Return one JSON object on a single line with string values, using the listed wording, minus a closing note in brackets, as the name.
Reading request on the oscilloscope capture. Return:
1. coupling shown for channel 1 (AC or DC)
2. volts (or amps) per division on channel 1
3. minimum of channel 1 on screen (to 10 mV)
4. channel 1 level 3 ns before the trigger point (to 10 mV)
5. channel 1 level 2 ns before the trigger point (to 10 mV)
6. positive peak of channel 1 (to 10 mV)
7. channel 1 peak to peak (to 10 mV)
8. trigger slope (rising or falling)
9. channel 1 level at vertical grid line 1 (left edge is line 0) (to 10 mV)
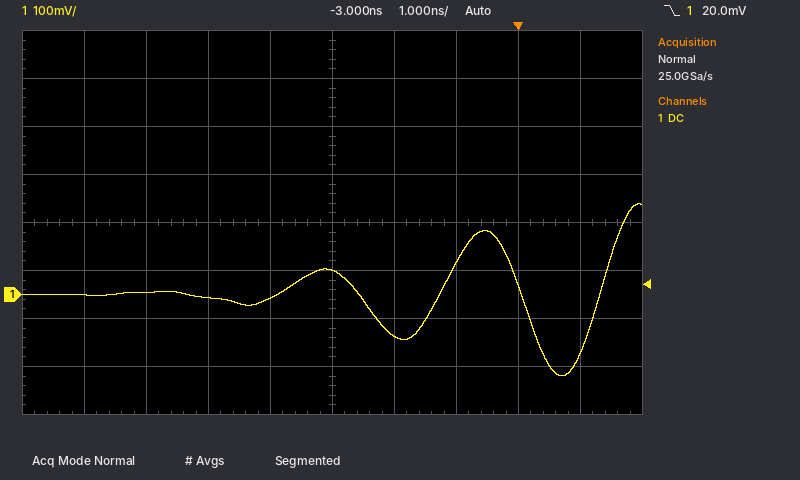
{"coupling shown for channel 1": "DC", "volts (or amps) per division on channel 1": "100 mV", "minimum of channel 1 on screen": "-170 mV", "channel 1 level 3 ns before the trigger point": "50 mV", "channel 1 level 2 ns before the trigger point": "-90 mV", "positive peak of channel 1": "190 mV", "channel 1 peak to peak": "360 mV", "trigger slope": "falling", "channel 1 level at vertical grid line 1 (left edge is line 0)": "0 mV"}
